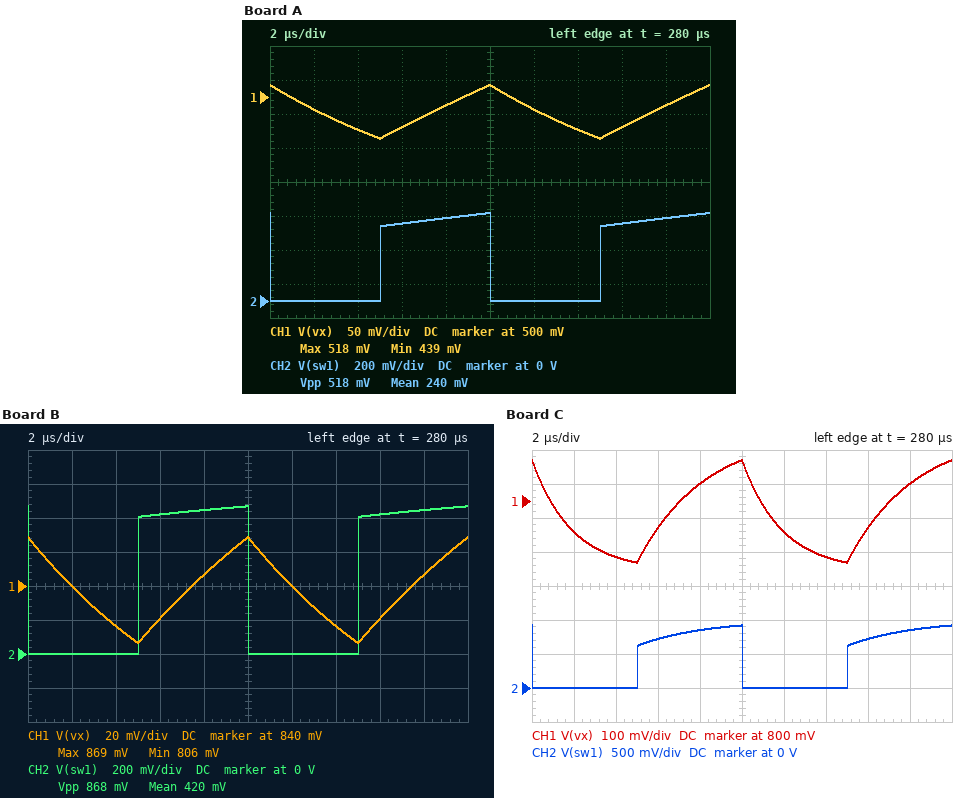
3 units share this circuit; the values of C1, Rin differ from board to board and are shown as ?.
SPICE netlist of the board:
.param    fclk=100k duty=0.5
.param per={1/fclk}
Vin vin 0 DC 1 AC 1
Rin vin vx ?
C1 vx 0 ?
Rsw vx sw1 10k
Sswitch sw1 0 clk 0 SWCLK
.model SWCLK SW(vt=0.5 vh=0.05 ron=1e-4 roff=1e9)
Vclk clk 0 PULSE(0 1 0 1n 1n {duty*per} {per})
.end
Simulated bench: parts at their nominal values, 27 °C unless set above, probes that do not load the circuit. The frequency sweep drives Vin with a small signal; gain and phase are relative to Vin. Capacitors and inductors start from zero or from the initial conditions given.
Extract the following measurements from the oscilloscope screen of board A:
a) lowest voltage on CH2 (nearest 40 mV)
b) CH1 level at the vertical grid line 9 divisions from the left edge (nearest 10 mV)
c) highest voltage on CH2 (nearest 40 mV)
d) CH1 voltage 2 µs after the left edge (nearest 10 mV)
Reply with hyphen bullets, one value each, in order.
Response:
- 0 V
- 490 mV
- 520 mV
- 480 mV
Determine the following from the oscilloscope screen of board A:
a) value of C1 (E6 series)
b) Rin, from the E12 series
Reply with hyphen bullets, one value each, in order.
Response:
- 1.5 nF
- 22 kΩ
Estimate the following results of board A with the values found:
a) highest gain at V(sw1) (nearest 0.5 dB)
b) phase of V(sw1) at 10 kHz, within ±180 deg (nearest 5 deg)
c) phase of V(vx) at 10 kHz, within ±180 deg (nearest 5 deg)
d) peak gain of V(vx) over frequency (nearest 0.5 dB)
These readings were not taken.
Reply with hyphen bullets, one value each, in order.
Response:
- 0 dB
- -65 deg
- -65 deg
- 0 dB
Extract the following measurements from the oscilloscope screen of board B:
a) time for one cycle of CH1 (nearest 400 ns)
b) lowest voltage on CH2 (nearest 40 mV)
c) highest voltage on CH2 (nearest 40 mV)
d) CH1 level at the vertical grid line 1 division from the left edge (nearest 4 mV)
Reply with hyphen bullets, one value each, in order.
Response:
- 10.0 µs
- 0 V
- 880 mV
- 840 mV
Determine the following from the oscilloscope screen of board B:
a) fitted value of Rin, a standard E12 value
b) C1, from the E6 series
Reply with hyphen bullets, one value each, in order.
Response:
- 3.9 kΩ
- 3.3 nF
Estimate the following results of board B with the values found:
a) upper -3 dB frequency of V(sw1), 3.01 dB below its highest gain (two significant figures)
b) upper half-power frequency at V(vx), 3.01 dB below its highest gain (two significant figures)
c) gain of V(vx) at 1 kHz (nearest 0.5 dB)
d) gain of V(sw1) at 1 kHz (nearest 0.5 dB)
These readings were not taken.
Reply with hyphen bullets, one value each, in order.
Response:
- 12 kHz
- 12 kHz
- 0 dB
- 0 dB
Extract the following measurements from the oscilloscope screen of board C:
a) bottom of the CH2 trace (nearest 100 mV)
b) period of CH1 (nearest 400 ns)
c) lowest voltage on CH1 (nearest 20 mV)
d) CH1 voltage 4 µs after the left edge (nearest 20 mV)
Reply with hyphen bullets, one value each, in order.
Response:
- 0 V
- 10.0 µs
- 620 mV
- 640 mV
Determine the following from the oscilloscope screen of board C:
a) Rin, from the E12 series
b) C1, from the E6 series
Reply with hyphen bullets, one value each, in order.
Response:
- 6.8 kΩ
- 470 pF
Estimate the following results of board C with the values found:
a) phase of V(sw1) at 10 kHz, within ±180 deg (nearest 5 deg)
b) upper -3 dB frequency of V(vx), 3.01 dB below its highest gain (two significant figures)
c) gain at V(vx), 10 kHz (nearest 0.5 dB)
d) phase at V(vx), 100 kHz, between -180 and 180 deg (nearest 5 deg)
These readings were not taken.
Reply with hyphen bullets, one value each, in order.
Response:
- -10 deg
- 50 kHz
- 0 dB
- -65 deg
